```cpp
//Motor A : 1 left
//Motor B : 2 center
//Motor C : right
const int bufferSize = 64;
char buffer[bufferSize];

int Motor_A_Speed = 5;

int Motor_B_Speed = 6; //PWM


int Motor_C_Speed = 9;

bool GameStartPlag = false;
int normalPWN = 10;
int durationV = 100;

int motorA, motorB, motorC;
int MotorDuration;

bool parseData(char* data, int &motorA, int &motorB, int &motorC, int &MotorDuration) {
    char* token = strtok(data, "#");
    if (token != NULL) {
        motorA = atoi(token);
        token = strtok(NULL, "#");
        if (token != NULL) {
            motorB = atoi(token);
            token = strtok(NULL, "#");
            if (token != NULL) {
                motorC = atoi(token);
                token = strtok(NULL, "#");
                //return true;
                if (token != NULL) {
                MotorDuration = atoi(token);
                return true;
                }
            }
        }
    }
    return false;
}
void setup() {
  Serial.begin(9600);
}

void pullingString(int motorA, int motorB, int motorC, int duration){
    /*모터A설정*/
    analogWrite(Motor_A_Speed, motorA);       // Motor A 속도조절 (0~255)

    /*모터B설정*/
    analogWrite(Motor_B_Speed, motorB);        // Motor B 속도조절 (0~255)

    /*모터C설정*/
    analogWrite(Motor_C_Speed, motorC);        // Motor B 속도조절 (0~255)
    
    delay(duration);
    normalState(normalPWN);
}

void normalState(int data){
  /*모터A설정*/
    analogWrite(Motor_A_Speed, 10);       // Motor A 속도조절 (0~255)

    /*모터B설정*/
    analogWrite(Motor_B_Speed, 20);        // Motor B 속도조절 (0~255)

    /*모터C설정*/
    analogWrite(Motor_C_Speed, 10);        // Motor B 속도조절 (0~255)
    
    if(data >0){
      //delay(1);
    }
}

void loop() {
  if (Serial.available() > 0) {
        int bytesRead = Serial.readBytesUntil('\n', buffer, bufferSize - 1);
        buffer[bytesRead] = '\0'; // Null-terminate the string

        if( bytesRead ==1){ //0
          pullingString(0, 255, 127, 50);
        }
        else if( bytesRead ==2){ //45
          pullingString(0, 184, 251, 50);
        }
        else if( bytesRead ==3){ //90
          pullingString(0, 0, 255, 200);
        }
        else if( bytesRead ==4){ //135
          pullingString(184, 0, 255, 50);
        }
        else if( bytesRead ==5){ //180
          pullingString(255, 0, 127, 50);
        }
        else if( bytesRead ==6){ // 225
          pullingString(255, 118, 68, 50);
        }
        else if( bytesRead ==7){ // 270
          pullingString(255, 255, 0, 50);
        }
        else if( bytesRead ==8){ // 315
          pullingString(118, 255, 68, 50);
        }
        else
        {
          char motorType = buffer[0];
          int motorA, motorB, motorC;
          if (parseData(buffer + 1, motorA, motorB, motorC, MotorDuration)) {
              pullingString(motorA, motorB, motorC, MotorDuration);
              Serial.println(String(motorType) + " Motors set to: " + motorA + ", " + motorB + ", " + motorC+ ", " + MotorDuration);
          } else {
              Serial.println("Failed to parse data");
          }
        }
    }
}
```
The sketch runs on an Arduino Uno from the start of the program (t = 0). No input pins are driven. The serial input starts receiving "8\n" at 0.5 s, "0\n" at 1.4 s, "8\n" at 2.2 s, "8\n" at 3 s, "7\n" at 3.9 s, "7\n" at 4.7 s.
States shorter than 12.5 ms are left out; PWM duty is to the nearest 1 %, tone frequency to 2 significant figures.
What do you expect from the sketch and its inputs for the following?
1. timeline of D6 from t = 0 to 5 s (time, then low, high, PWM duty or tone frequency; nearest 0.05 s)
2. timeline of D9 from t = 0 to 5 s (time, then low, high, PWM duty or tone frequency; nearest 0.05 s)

0.5 s high; 0.55 s PWM 8 %; 1.4 s high; 1.45 s PWM 8 %; 2.2 s high; 2.25 s PWM 8 %; 3 s high; 3.05 s PWM 8 %; 3.9 s high; 3.95 s PWM 8 %; 4.7 s high; 4.75 s PWM 8 %
0.5 s PWM 50 %; 0.55 s PWM 4 %; 1.4 s PWM 50 %; 1.45 s PWM 4 %; 2.2 s PWM 50 %; 2.25 s PWM 4 %; 3 s PWM 50 %; 3.05 s PWM 4 %; 3.9 s PWM 50 %; 3.95 s PWM 4 %; 4.7 s PWM 50 %; 4.75 s PWM 4 %
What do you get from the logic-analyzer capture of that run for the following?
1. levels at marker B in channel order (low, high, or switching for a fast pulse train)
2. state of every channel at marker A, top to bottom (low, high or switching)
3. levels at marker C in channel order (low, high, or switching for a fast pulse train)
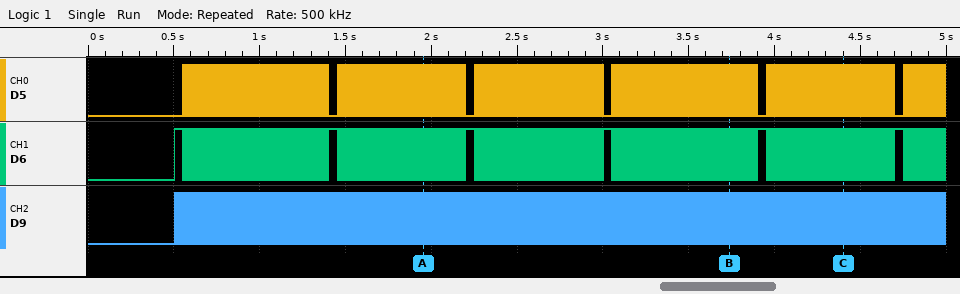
D5 switching, D6 switching, D9 switching
D5 switching, D6 switching, D9 switching
D5 switching, D6 switching, D9 switching
